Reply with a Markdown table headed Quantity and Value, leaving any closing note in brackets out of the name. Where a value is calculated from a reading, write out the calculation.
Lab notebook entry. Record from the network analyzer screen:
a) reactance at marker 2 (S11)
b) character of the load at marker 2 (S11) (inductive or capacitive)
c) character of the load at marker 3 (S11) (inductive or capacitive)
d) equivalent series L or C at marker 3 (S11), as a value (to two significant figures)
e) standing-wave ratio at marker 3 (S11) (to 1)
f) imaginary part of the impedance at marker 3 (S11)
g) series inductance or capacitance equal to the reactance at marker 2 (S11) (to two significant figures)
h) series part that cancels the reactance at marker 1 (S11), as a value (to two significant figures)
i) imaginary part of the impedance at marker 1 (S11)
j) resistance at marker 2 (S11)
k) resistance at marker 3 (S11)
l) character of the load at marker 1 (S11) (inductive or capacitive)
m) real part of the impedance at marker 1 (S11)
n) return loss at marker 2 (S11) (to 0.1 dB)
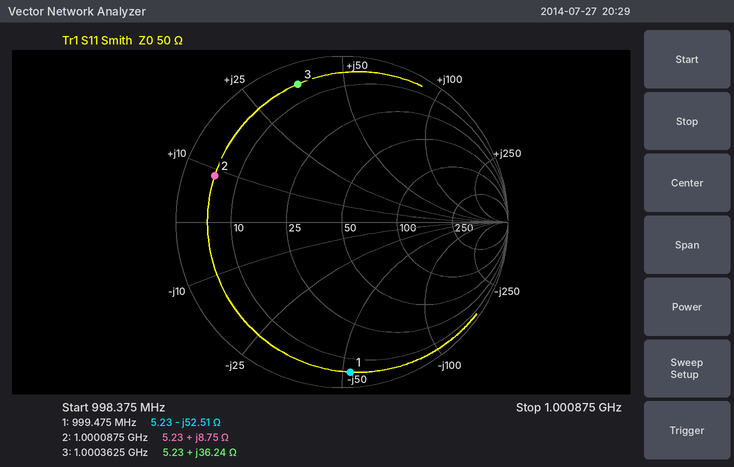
| Quantity | Value |
|---|---|
| reactance at marker 2 | +8.75 Ω |
| character of the load at marker 2 (S11) | inductive |
| character of the load at marker 3 (S11) | inductive |
| equivalent series L or C at marker 3 (S11), as a value | L = 36.24 Ω/(2π × 1.0003625 GHz) ≈ 5.8 nH |
| standing-wave ratio at marker 3 (S11) | 15 |
| imaginary part of the impedance at marker 3 | +36.24 Ω |
| series inductance or capacitance equal to the reactance at marker 2 (S11) | L = 8.75 Ω/(2π × 1.0000875 GHz) ≈ 1.4 nH |
| series part that cancels the reactance at marker 1 (S11), as a value | L = 52.51 Ω/(2π × 999.475 MHz) ≈ 8.4 nH |
| imaginary part of the impedance at marker 1 | -52.51 Ω |
| resistance at marker 2 | 5.23 Ω |
| resistance at marker 3 | 5.23 Ω |
| character of the load at marker 1 (S11) | capacitive |
| real part of the impedance at marker 1 | 5.23 Ω |
| return loss at marker 2 (S11) | 1.8 dB |
